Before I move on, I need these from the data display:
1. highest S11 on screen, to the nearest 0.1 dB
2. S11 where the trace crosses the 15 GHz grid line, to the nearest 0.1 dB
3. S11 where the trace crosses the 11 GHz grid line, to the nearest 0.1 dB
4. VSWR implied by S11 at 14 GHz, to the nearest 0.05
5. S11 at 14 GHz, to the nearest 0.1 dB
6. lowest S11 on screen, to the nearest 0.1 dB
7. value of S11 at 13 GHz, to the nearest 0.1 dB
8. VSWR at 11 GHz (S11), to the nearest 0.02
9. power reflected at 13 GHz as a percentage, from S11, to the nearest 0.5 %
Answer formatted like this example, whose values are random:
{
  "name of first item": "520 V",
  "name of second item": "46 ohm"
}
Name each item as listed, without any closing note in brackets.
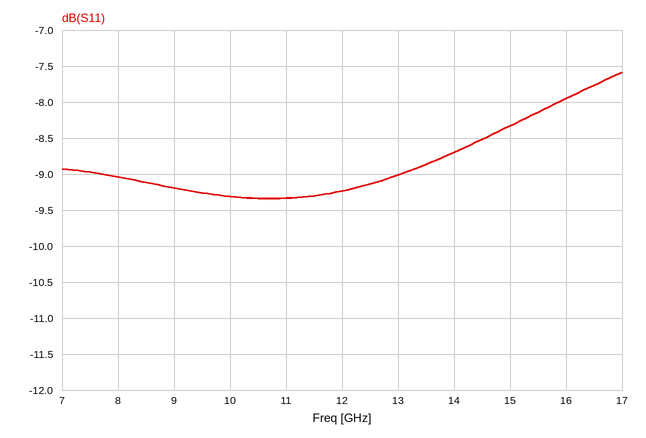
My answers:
{
  "highest S11 on screen, to the nearest 0.1 dB": "-7.6 dB",
  "S11 where the trace crosses the 15 GHz grid line, to the nearest 0.1 dB": "-8.3 dB",
  "S11 where the trace crosses the 11 GHz grid line, to the nearest 0.1 dB": "-9.3 dB",
  "VSWR implied by S11 at 14 GHz, to the nearest 0.05": "2.15",
  "S11 at 14 GHz, to the nearest 0.1 dB": "-8.7 dB",
  "lowest S11 on screen, to the nearest 0.1 dB": "-9.3 dB",
  "value of S11 at 13 GHz, to the nearest 0.1 dB": "-9.0 dB",
  "VSWR at 11 GHz (S11), to the nearest 0.02": "2.04",
  "power reflected at 13 GHz as a percentage, from S11, to the nearest 0.5 %": "12.5 %"
}
